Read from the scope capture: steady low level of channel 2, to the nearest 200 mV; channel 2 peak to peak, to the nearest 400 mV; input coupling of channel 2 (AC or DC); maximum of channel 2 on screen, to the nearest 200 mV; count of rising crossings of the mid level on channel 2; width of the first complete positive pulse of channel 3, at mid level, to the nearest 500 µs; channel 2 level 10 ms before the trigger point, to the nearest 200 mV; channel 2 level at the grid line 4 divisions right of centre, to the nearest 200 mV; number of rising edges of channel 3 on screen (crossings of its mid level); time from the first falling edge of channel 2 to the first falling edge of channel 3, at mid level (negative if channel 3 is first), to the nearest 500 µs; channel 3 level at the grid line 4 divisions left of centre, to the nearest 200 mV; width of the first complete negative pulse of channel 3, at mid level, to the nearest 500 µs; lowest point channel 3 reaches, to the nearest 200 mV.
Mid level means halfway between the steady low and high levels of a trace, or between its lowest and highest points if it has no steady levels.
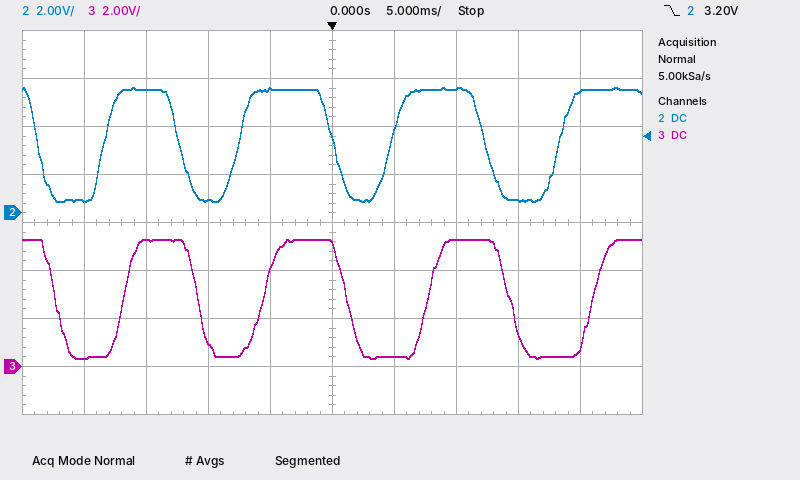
600 mV
4.8 V
DC
5.2 V
4
6.0 ms
600 mV
5.0 V
4
+1.5 ms
400 mV
5.5 ms
400 mV
